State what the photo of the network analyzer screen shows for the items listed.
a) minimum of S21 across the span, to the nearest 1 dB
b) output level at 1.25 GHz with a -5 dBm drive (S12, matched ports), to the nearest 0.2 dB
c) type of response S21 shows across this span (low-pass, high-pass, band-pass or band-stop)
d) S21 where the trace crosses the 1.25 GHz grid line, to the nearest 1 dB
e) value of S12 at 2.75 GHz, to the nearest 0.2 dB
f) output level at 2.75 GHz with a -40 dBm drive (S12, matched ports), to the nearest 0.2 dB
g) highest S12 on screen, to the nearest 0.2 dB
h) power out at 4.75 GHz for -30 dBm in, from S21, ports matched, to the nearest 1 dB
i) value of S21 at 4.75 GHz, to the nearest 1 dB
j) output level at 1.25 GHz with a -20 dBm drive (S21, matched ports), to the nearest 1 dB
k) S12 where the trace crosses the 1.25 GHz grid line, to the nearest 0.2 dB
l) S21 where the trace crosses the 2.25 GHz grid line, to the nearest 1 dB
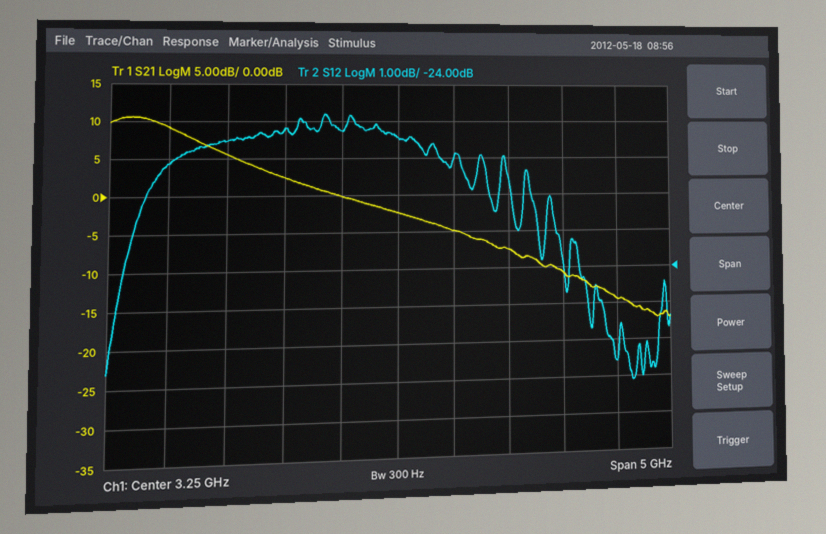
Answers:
-17 dB
-26.2 dBm
low-pass
9 dB
-20.2 dB
-60.2 dBm
-19.8 dB
-41 dBm
-11 dB
-11 dBm
-21.2 dB
2 dB
